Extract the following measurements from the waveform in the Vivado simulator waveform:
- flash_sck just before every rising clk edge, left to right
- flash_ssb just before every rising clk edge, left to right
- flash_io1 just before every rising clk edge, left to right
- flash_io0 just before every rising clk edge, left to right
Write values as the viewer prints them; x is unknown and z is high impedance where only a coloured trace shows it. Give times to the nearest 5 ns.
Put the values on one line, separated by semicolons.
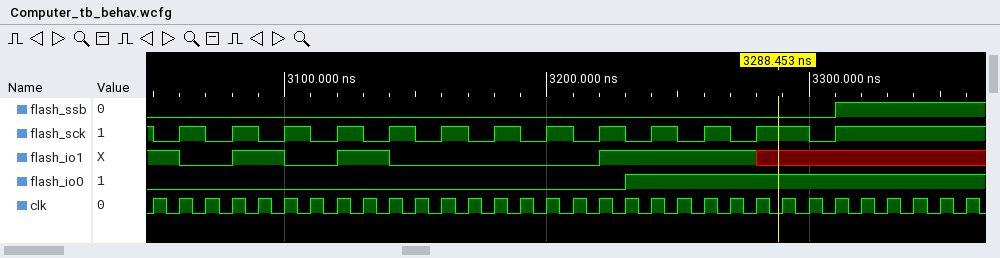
1 0 1 0 1 0 1 0 1 0 1 0 1 0 1 0 1 0 1 0 1 0 1 0 1 1 0 1 1 1 1 1; 0 0 0 0 0 0 0 0 0 0 0 0 0 0 0 0 0 0 0 0 0 0 0 0 0 0 0 1 1 1 1 1; 1 1 0 0 1 1 0 0 1 1 0 0 0 0 0 0 0 0 1 1 1 1 1 1 x x x x x x x x; 0 0 0 0 0 0 0 0 0 0 0 0 0 0 0 0 0 0 0 1 1 1 1 1 1 1 1 1 1 1 1 1
